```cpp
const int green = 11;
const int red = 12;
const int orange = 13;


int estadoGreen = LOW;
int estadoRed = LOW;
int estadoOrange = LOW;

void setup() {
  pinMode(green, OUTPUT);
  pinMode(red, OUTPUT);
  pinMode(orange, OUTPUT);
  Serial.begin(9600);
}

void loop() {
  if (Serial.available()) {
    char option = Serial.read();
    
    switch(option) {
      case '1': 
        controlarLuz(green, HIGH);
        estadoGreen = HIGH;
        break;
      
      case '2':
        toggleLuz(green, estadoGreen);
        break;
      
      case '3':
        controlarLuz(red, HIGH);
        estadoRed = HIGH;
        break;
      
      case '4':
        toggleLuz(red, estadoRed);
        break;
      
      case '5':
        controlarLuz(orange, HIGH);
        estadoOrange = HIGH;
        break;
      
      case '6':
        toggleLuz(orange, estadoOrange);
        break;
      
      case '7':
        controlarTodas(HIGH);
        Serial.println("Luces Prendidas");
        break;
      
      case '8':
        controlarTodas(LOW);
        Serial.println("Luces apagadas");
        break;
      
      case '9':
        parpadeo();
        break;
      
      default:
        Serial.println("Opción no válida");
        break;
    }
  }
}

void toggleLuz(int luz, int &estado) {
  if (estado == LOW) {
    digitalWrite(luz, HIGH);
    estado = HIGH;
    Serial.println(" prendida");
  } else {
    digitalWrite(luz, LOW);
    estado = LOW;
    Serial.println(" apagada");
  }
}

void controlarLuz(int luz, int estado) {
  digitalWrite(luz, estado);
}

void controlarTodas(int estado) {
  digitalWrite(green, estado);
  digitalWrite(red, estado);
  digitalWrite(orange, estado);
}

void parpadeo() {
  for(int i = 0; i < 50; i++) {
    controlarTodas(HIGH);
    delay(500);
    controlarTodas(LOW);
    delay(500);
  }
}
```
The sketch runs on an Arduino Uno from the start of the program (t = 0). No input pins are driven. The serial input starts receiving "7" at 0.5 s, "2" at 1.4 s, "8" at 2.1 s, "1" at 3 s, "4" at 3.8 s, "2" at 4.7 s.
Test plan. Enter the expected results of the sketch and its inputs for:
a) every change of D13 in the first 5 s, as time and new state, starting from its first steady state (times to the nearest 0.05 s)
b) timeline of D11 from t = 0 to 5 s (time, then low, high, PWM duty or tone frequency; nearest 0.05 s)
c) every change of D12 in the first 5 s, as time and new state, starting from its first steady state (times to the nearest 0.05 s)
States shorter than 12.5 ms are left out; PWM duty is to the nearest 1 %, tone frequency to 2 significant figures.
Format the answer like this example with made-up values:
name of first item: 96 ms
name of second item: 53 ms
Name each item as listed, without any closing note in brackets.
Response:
every change of D13 in the first 5 s, as time and new state, starting from its first steady state: 0 s low; 0.5 s high; 2.1 s low
timeline of D11 from t = 0 to 5 s: 0 s low; 0.5 s high; 2.1 s low; 3 s high; 4.7 s low
every change of D12 in the first 5 s, as time and new state, starting from its first steady state: 0 s low; 0.5 s high; 2.1 s low; 3.8 s high
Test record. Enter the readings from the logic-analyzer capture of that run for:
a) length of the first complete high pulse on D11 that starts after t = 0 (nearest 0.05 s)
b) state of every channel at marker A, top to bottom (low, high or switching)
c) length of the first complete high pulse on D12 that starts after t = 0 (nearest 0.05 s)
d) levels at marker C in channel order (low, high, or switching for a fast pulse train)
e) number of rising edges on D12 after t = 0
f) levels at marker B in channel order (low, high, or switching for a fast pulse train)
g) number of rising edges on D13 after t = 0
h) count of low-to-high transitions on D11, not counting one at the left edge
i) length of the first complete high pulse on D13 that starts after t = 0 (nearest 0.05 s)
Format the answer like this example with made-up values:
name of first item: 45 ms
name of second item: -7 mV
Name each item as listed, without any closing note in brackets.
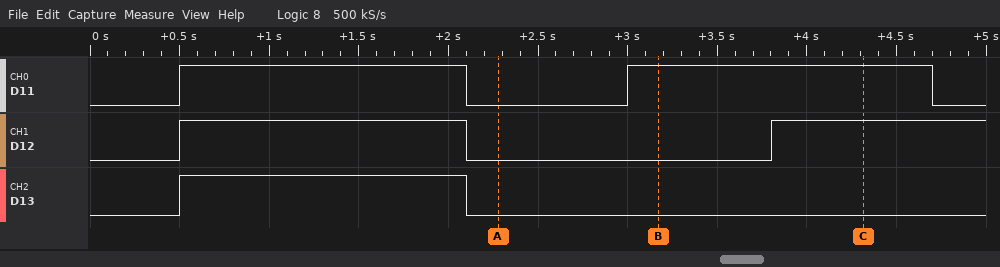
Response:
length of the first complete high pulse on D11 that starts after t = 0: 1.60 s
state of every channel at marker A, top to bottom: D11 low, D12 low, D13 low
length of the first complete high pulse on D12 that starts after t = 0: 1.60 s
levels at marker C in channel order: D11 high, D12 high, D13 low
number of rising edges on D12 after t = 0: 2
levels at marker B in channel order: D11 high, D12 low, D13 low
number of rising edges on D13 after t = 0: 1
count of low-to-high transitions on D11, not counting one at the left edge: 2
length of the first complete high pulse on D13 that starts after t = 0: 1.60 s
